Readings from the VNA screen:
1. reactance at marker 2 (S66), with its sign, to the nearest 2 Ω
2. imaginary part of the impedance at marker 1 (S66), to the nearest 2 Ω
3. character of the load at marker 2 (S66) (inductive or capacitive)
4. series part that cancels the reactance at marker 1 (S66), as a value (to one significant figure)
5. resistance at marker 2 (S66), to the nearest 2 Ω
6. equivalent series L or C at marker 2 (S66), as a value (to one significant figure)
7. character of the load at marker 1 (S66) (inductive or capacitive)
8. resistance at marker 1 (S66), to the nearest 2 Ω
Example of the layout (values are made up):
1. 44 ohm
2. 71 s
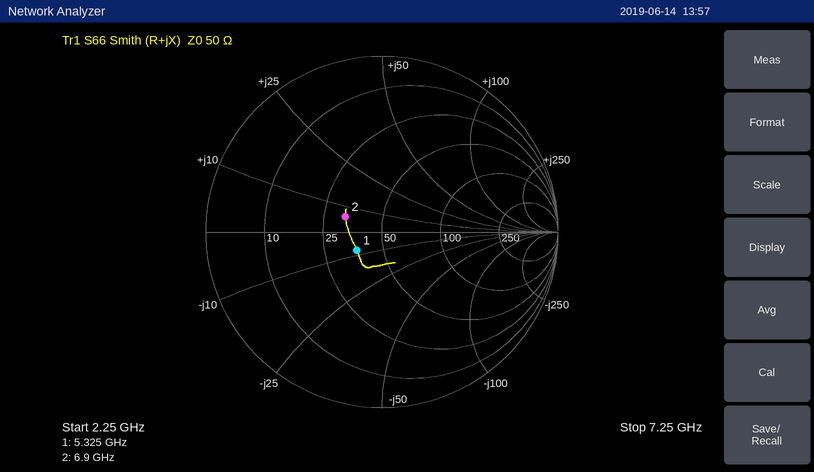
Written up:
1. +6 Ω
2. -8 Ω
3. inductive
4. 200 pH
5. 32 Ω
6. 100 pH
7. capacitive
8. 36 Ω
